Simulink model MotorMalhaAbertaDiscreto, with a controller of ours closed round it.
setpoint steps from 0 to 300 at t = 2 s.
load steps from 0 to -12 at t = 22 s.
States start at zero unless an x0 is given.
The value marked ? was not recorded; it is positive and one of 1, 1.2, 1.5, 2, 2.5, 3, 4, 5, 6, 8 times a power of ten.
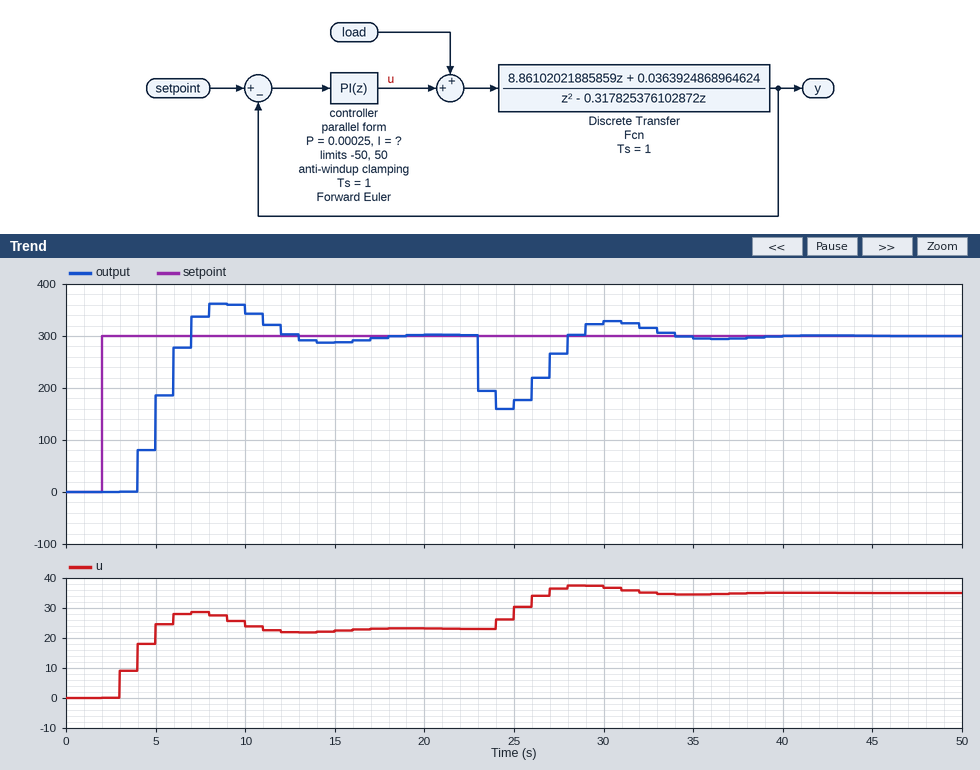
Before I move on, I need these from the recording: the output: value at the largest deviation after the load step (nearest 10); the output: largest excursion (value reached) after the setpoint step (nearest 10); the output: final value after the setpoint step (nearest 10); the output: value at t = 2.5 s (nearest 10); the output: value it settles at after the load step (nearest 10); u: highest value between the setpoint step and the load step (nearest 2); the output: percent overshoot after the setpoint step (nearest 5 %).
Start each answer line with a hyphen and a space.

- 160
- 360
- 300
- 0
- 300
- 28
- 20 %
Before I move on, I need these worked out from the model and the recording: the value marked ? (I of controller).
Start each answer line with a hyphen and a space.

- 0.03
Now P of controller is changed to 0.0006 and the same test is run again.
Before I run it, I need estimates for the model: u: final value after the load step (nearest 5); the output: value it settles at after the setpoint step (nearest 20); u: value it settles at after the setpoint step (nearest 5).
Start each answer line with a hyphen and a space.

- 35
- 300
- 25
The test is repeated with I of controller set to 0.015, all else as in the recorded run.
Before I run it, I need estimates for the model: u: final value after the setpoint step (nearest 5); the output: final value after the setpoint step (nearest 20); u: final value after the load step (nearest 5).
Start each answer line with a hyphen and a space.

- 25
- 300
- 35
